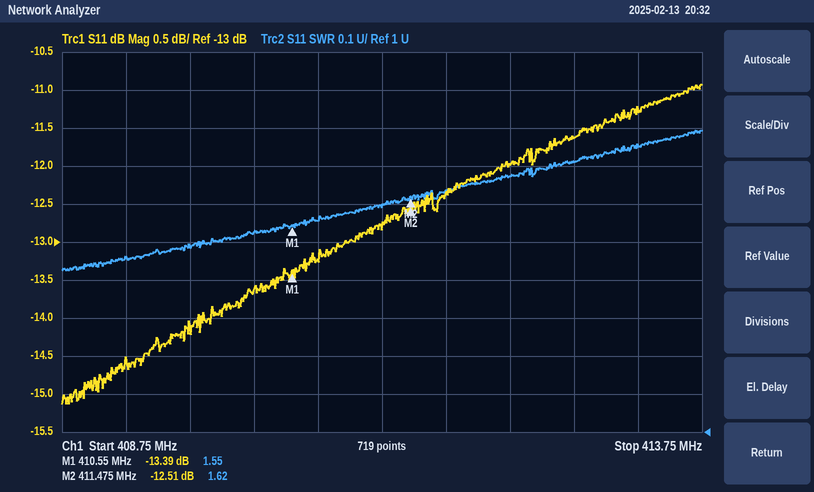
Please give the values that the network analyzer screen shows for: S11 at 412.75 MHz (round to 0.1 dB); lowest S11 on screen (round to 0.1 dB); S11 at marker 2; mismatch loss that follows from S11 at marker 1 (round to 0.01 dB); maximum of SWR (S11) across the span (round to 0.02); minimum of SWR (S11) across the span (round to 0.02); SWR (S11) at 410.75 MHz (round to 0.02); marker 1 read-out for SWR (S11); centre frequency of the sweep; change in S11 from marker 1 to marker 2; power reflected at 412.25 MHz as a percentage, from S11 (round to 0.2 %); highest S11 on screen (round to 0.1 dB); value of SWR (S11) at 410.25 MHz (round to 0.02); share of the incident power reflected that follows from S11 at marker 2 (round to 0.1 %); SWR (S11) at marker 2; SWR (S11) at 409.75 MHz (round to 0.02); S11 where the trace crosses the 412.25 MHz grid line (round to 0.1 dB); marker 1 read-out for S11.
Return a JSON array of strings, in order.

["-11.6 dB", "-15.1 dB", "-12.51 dB", "0.20 dB", "1.80", "1.42", "1.56", "1.55", "411.25 MHz", "0.88 dB", "6.4 %", "-10.9 dB", "1.52", "5.6 %", "1.62", "1.48", "-12.0 dB", "-13.39 dB"]
